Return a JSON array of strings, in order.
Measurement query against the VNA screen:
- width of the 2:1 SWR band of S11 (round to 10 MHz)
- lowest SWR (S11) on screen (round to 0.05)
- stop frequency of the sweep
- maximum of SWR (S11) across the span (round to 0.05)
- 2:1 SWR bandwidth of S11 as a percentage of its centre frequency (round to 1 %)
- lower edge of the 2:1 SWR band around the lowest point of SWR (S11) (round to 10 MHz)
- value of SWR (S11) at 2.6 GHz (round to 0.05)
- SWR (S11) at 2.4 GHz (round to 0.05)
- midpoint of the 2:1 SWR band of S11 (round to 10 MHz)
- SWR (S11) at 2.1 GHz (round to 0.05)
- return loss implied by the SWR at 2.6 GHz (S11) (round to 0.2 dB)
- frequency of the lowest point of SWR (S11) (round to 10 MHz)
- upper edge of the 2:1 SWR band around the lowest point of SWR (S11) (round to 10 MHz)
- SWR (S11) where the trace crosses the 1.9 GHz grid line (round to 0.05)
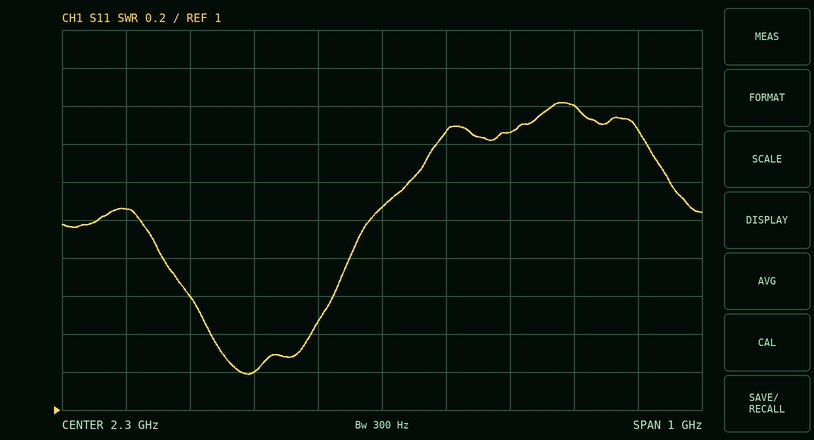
["360 MHz", "1.20", "2.8 GHz", "2.60", "17 %", "1.92 GHz", "2.60", "2.45", "2.10 GHz", "1.20", "7.0 dB", "2.09 GHz", "2.28 GHz", "2.05"]
